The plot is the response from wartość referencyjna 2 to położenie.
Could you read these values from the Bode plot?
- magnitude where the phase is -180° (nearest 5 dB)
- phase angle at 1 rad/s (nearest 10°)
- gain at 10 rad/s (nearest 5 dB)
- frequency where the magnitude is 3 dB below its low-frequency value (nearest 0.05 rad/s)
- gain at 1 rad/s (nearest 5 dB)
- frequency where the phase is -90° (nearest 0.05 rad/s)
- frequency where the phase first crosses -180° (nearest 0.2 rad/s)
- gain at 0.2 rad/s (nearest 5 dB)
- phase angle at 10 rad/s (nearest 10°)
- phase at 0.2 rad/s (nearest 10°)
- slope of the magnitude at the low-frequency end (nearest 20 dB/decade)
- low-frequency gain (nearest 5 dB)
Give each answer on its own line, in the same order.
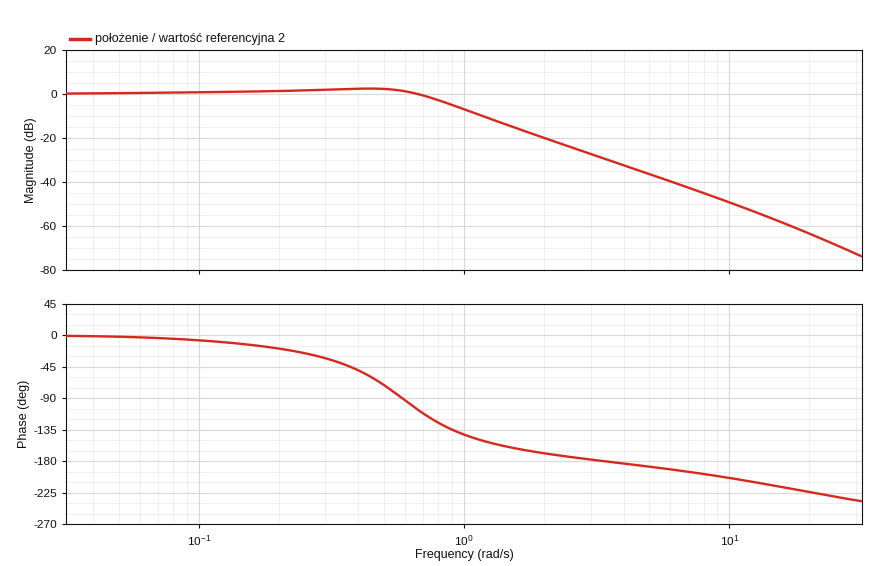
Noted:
-30 dB
-140°
-50 dB
0.80 rad/s
-5 dB
0.60 rad/s
3.4 rad/s
0 dB
-200°
-20°
0 dB/decade
0 dB
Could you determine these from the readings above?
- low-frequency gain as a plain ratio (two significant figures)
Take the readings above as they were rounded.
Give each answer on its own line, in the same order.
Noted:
1.0
